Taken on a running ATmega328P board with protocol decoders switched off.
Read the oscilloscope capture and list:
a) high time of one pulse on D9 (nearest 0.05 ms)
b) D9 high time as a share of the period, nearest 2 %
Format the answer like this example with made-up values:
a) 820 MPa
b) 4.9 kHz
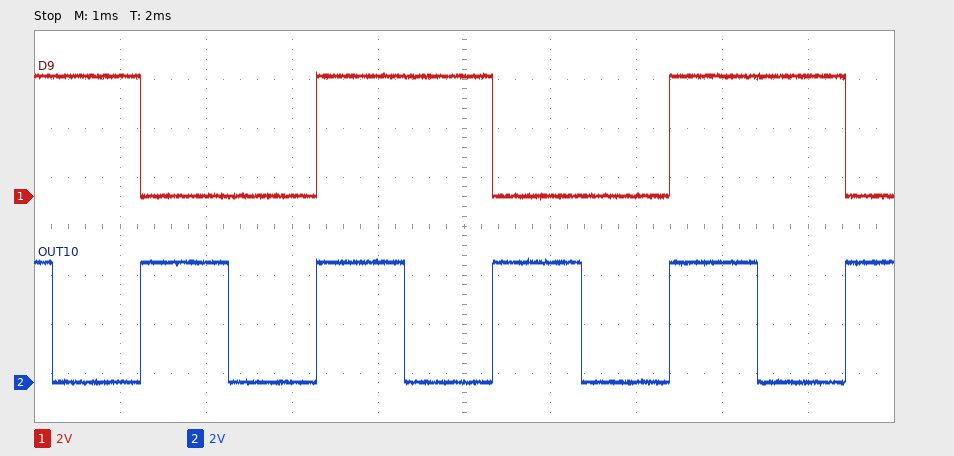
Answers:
a) 2.05 ms
b) 50 %
